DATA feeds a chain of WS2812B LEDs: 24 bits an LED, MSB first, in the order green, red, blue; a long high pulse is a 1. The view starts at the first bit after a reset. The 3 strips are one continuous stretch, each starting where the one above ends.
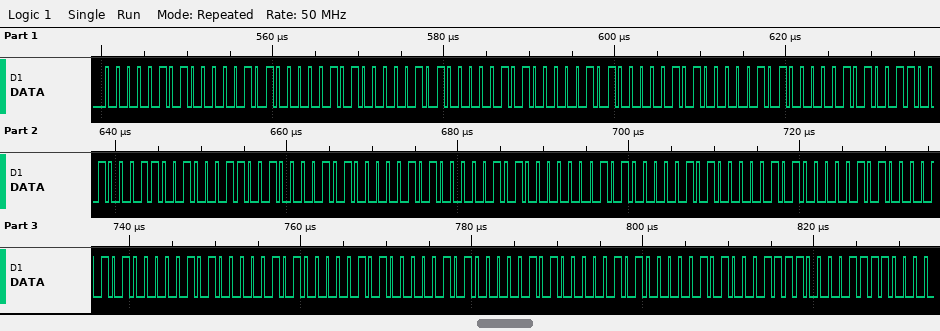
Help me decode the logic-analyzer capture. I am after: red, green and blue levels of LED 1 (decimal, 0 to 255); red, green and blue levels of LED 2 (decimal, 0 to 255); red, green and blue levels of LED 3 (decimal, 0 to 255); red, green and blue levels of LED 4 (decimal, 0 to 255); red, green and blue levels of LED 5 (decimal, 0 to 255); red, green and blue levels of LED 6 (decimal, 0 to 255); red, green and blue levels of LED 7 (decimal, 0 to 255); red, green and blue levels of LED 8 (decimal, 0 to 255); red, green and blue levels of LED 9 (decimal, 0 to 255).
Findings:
5, 5, 5
5, 5, 5
5, 5, 5
50, 50, 50
20, 20, 20
5, 5, 5
5, 5, 5
5, 5, 5
5, 5, 5
